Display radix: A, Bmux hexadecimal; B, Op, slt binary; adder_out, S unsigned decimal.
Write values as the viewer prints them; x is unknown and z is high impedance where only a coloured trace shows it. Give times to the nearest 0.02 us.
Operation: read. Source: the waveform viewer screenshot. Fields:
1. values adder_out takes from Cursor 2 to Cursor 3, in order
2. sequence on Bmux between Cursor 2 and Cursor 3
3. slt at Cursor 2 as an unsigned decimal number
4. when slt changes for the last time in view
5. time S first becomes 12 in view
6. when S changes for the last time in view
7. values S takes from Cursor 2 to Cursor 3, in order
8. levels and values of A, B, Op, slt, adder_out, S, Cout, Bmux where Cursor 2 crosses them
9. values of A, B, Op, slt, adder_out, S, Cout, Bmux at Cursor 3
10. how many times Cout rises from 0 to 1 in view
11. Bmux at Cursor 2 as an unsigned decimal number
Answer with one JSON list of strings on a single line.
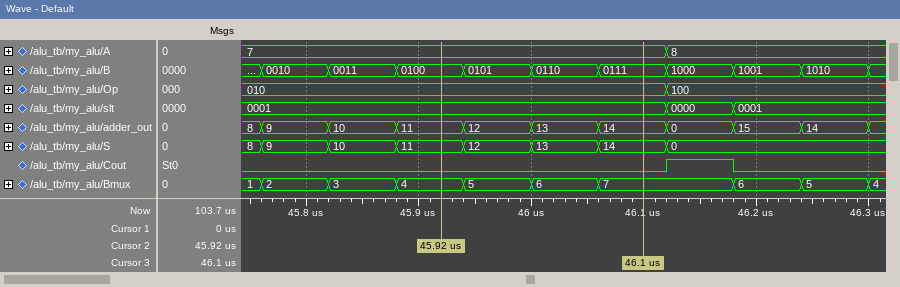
["11, 12, 13, 14", "4, 5, 6, 7", "1", "46.18 us", "45.94 us", "46.12 us", "11, 12, 13, 14", "A=7, B=0100, Op=010, slt=0001, adder_out=11, S=11, Cout=0, Bmux=4", "A=7, B=0111, Op=010, slt=0001, adder_out=14, S=14, Cout=0, Bmux=7", "1", "4"]
